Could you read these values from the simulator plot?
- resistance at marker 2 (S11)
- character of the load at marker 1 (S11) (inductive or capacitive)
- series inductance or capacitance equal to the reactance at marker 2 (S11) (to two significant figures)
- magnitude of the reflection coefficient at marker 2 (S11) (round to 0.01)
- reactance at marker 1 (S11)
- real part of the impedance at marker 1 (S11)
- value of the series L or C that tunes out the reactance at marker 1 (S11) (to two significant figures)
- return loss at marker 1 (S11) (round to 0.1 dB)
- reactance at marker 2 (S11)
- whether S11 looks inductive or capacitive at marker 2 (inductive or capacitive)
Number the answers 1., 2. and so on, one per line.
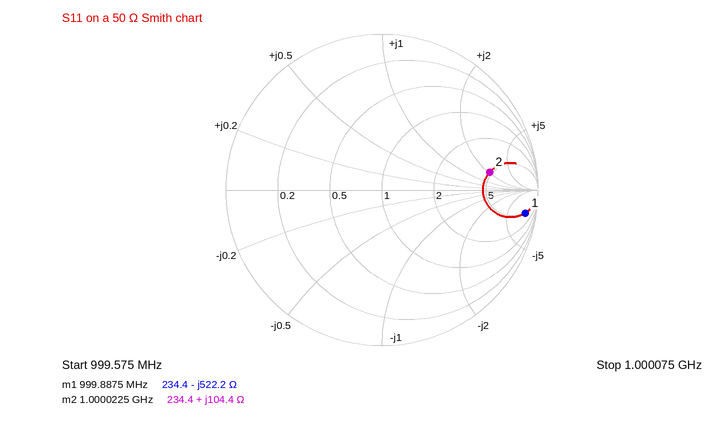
1. 234.4 Ω
2. capacitive
3. 17 nH
4. 0.70
5. -522.2 Ω
6. 234.4 Ω
7. 83 nH
8. 0.6 dB
9. +104.4 Ω
10. inductive
